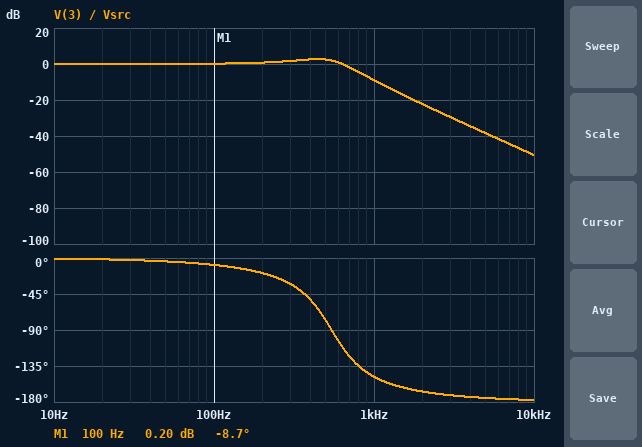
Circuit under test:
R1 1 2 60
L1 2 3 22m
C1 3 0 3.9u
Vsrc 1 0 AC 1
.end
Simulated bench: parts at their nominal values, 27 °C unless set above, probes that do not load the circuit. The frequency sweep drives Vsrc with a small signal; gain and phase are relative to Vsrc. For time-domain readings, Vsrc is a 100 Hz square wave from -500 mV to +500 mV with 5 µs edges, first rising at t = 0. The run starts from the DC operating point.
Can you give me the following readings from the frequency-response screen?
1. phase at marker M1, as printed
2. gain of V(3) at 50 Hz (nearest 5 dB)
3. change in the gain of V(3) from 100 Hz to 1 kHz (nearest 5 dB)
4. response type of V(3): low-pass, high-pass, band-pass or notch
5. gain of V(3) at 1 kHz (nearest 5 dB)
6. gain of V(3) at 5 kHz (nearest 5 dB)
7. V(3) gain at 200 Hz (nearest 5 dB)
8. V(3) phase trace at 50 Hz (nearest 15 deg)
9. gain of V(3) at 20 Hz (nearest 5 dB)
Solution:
-8.7 deg
0 dB
-10 dB
low-pass
-10 dB
-40 dB
0 dB
0 deg
0 dB
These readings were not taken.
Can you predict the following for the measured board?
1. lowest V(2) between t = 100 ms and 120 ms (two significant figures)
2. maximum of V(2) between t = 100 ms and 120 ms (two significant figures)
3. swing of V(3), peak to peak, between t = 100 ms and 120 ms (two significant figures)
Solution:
-620 mV
620 mV
1.5 V
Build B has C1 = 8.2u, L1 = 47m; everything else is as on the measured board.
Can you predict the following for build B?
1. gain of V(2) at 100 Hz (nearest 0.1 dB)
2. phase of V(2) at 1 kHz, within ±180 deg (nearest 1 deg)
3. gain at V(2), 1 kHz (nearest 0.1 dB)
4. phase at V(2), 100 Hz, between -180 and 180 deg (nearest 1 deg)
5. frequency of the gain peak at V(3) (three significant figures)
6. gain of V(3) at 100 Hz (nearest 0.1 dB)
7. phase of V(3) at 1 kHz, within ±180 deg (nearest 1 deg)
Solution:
-0.5 dB
12 deg
-0.2 dB
-20 deg
212 Hz
0.9 dB
-168 deg
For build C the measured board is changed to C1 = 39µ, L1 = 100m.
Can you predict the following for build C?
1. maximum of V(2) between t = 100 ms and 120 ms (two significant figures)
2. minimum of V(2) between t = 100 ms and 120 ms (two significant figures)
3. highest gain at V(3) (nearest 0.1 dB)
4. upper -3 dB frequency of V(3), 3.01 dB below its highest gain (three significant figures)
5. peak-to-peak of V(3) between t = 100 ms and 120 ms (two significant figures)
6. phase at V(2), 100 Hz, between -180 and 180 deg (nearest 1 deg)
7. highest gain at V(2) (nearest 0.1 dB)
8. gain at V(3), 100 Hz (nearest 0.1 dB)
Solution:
840 mV
-840 mV
0.4 dB
90.2 Hz
850 mV
70 deg
0 dB
-3.9 dB
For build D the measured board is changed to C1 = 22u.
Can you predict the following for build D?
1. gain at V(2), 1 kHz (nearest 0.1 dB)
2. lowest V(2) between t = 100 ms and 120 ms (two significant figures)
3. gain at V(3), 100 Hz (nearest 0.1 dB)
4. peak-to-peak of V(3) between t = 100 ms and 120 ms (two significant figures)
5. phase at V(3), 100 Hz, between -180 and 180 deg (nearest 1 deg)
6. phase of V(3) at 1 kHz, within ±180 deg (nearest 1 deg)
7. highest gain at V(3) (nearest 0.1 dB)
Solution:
-0.8 dB
-500 mV
-1.3 dB
1.0 V
-46 deg
-155 deg
0 dB
